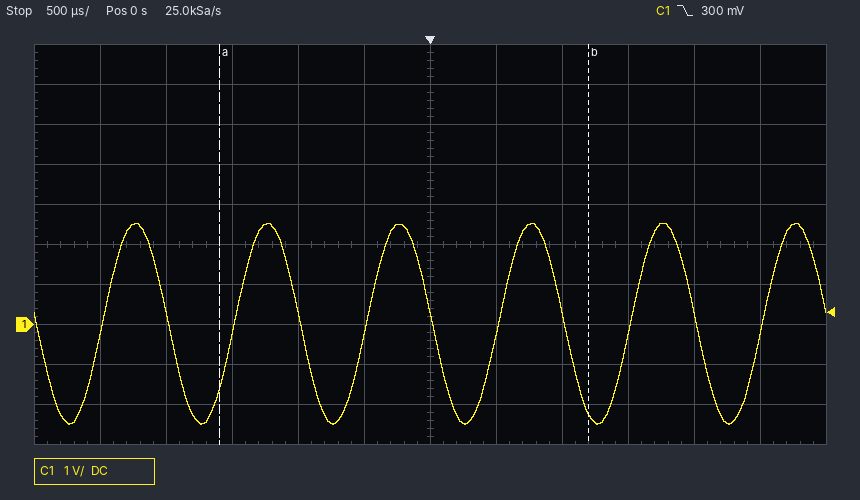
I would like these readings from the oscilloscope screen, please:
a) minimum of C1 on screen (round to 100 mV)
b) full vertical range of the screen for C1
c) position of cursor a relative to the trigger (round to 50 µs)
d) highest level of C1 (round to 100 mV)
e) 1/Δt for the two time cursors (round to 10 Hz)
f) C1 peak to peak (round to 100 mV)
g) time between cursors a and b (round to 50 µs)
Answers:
-2.5 V
10 V
-1.60 ms
2.5 V
360 Hz
5.0 V
2.80 ms
